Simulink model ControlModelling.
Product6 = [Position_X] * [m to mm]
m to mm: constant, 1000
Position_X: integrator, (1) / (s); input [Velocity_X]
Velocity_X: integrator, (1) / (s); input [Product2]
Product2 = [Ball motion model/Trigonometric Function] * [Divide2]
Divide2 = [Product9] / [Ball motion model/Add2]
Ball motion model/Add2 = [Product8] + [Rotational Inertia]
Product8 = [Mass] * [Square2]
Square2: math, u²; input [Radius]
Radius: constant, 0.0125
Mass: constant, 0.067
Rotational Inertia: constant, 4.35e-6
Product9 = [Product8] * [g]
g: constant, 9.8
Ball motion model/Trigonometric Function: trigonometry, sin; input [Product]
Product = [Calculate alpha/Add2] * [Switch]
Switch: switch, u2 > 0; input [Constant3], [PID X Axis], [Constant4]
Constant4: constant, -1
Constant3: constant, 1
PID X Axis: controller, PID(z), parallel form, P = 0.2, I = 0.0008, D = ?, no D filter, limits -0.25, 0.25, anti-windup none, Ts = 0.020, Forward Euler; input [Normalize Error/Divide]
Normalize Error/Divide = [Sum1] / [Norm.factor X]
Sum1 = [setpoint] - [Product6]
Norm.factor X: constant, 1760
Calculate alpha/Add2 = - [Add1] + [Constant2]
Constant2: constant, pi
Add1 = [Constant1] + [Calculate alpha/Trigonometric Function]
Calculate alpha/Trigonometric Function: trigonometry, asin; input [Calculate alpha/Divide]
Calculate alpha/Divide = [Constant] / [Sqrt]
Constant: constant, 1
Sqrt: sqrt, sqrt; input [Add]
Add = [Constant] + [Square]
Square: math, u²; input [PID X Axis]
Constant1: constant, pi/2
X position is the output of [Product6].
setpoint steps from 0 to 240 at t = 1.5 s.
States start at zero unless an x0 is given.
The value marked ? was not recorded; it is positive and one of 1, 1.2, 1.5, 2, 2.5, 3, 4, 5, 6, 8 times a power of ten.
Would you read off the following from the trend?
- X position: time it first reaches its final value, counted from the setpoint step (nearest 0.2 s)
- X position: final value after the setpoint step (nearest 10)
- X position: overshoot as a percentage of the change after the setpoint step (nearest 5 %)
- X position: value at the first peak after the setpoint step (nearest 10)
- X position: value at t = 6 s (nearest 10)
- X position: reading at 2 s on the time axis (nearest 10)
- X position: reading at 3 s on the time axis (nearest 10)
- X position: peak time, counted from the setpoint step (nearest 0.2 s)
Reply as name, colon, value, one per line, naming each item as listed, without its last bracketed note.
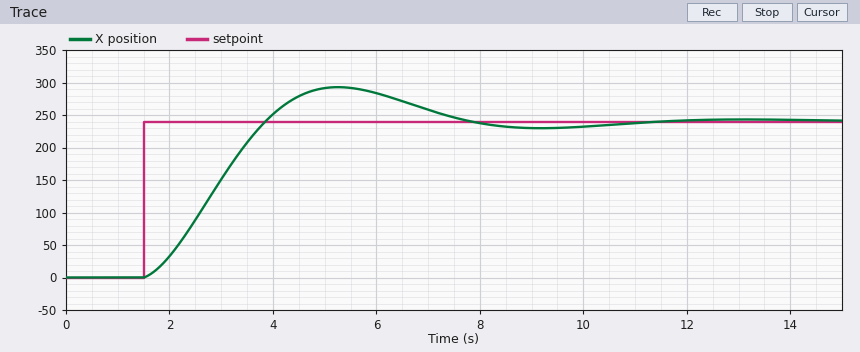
X position: time it first reaches its final value, counted from the setpoint step: 2.4 s
X position: final value after the setpoint step: 240
X position: overshoot as a percentage of the change after the setpoint step: 20 %
X position: value at the first peak after the setpoint step: 290
X position: value at t = 6 s: 280
X position: reading at 2 s on the time axis: 30
X position: reading at 3 s on the time axis: 150
X position: peak time, counted from the setpoint step: 3.8 s
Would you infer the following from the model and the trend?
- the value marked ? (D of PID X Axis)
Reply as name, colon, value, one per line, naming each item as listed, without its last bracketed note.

the value marked ?: 0.2
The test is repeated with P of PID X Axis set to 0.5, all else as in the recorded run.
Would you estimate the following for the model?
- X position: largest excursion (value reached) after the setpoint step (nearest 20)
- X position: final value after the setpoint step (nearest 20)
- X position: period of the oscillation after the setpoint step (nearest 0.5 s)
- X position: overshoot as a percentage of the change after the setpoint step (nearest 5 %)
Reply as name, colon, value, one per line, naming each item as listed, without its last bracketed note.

X position: largest excursion (value reached) after the setpoint step: 340
X position: final value after the setpoint step: 240
X position: period of the oscillation after the setpoint step: 4.5 s
X position: overshoot as a percentage of the change after the setpoint step: 40 %
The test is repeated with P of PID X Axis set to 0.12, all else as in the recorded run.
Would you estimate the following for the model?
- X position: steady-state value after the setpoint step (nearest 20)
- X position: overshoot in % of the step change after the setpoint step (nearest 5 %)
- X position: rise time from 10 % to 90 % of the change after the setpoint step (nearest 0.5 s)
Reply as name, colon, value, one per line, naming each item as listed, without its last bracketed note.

X position: steady-state value after the setpoint step: 240
X position: overshoot in % of the step change after the setpoint step: 10 %
X position: rise time from 10 % to 90 % of the change after the setpoint step: 2.5 s
